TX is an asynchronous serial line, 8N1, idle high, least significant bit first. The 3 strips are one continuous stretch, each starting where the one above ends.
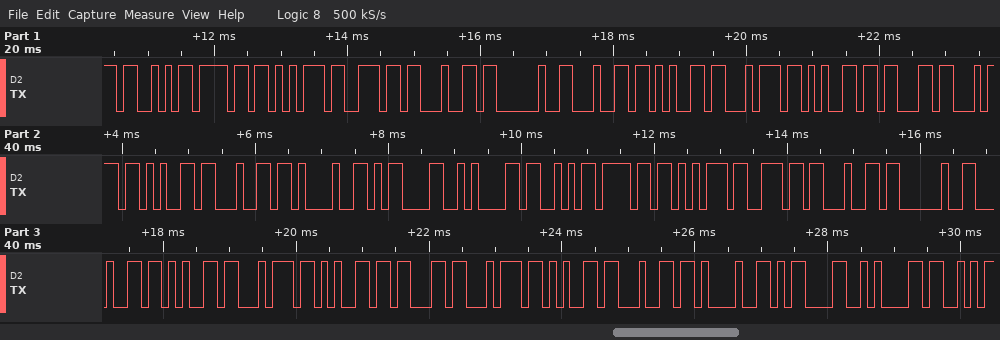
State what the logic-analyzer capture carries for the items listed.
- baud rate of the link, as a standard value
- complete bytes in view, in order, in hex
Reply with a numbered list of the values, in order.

1. 9600 baud
2. 53 6F 75 6E 64 20 64 65 74 65 63 74 65 64 21 0D 0A 53 6F 75 6E 64 20 64 65 74 65 63 74 65 64 21 0D 0A 53
